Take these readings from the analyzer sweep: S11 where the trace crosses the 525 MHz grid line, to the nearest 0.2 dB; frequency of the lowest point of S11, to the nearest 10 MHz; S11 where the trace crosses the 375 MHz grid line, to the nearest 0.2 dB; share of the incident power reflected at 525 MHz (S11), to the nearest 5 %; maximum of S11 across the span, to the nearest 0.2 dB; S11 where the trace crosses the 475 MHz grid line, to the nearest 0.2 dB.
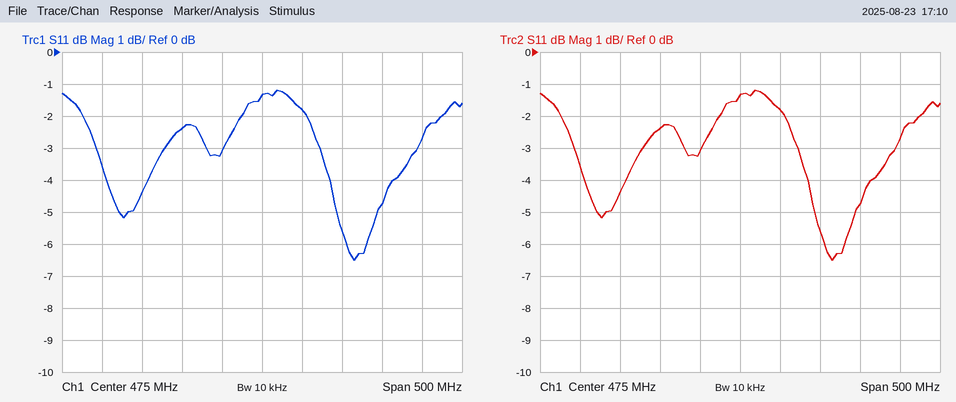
-1.8 dB
590 MHz
-2.4 dB
65 %
-1.2 dB
-1.4 dB
